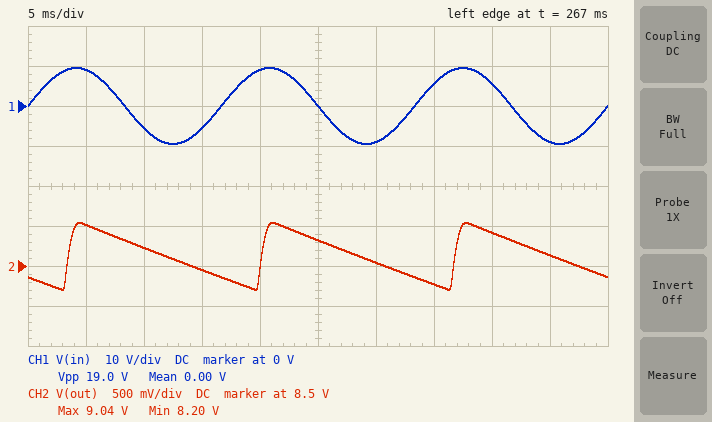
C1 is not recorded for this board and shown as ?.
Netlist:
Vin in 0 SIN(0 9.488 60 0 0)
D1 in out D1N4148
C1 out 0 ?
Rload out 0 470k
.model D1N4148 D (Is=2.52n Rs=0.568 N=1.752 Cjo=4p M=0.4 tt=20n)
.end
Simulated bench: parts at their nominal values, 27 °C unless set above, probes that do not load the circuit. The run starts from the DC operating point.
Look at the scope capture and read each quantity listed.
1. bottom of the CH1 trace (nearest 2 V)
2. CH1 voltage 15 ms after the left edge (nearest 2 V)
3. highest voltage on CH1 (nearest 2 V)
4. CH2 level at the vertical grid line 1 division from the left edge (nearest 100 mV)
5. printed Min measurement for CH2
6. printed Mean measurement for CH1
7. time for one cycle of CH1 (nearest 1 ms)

-10 V
-6 V
10 V
9.0 V
8.20 V
0.00 V
17 ms
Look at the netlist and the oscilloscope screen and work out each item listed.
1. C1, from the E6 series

330 nF
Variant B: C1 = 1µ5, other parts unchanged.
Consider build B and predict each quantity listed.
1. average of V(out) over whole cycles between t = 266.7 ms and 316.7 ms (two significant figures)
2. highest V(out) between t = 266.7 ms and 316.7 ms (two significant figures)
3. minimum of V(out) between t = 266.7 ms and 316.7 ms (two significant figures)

8.9 V
9.0 V
8.8 V
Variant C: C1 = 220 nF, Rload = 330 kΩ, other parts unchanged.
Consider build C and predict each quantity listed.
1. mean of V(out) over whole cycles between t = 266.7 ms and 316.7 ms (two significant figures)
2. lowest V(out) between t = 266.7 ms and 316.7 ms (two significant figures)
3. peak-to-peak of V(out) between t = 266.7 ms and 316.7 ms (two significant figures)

8.2 V
7.4 V
1.7 V
